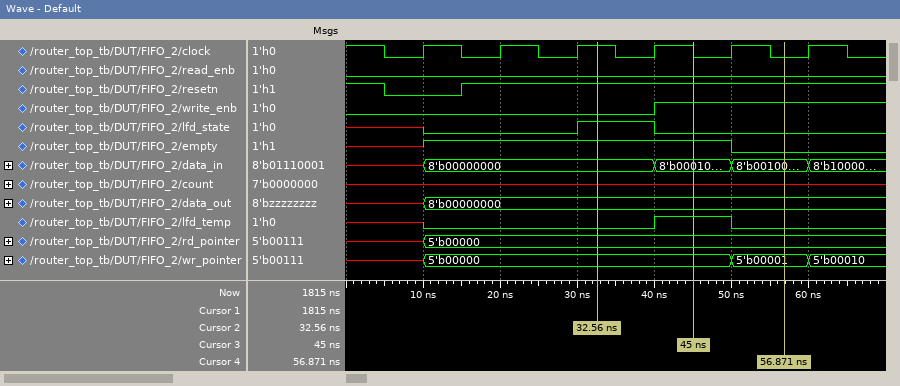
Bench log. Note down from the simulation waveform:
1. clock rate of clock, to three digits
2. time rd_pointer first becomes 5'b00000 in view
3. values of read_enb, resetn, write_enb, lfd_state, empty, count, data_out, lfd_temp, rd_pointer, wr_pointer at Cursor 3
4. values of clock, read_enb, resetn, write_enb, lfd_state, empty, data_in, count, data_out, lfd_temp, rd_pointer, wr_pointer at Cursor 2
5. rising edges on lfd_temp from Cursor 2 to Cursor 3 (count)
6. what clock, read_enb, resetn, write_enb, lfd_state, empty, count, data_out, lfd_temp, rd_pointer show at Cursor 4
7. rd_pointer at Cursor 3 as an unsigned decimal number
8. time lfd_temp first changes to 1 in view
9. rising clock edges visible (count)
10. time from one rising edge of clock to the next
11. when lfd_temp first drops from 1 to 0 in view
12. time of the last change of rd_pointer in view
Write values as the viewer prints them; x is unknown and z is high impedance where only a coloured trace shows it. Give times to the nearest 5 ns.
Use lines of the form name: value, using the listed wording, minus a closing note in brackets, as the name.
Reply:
clock rate of clock, to three digits: 100 MHz
time rd_pointer first becomes 5'b00000 in view: 10 ns
values of read_enb, resetn, write_enb, lfd_state, empty, count, data_out, lfd_temp, rd_pointer, wr_pointer at Cursor 3: read_enb=0, resetn=1, write_enb=1, lfd_state=0, empty=1, count=x, data_out=8'b00000000, lfd_temp=1, rd_pointer=5'b00000, wr_pointer=5'b00000
values of clock, read_enb, resetn, write_enb, lfd_state, empty, data_in, count, data_out, lfd_temp, rd_pointer, wr_pointer at Cursor 2: clock=1, read_enb=0, resetn=1, write_enb=0, lfd_state=1, empty=1, data_in=8'b00000000, count=x, data_out=8'b00000000, lfd_temp=0, rd_pointer=5'b00000, wr_pointer=5'b00000
rising edges on lfd_temp from Cursor 2 to Cursor 3: 1
what clock, read_enb, resetn, write_enb, lfd_state, empty, count, data_out, lfd_temp, rd_pointer show at Cursor 4: clock=0, read_enb=0, resetn=1, write_enb=1, lfd_state=0, empty=0, count=x, data_out=8'b00000000, lfd_temp=0, rd_pointer=5'b00000
rd_pointer at Cursor 3 as an unsigned decimal number: 0
time lfd_temp first changes to 1 in view: 40 ns
rising clock edges visible: 6
time from one rising edge of clock to the next: 10 ns
when lfd_temp first drops from 1 to 0 in view: 50 ns
time of the last change of rd_pointer in view: 10 ns
